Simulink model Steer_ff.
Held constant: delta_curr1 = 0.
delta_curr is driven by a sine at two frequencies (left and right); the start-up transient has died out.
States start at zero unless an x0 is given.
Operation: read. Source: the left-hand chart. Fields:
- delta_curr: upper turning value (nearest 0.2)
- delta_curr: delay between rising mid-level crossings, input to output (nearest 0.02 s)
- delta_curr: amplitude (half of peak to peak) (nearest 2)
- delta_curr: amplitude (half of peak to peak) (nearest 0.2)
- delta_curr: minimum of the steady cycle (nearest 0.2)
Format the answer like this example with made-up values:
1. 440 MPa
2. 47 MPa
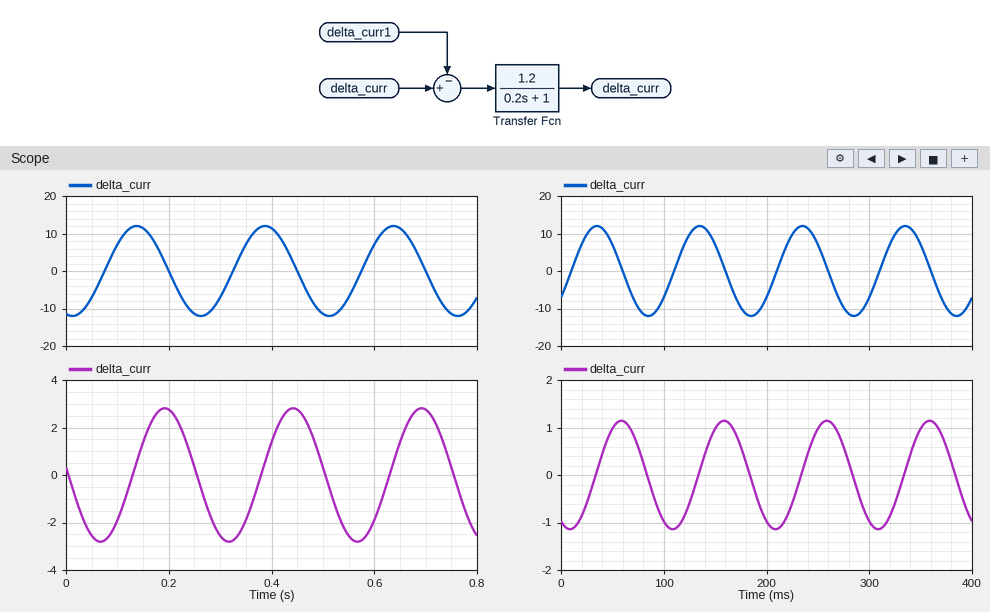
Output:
1. 2.8
2. 0.06 s
3. 12
4. 2.8
5. -2.8
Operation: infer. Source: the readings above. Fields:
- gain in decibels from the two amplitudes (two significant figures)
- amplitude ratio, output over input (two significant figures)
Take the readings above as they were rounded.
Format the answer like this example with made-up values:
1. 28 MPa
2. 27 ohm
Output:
1. -13 dB
2. 0.23
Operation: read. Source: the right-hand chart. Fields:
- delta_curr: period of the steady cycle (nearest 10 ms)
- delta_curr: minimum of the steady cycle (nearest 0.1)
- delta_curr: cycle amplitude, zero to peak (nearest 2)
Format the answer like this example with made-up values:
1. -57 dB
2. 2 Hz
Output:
1. 100 ms
2. -1.1
3. 12
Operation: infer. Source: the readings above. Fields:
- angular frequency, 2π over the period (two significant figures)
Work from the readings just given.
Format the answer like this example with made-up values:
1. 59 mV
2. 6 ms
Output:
1. 0.063 rad/ms
